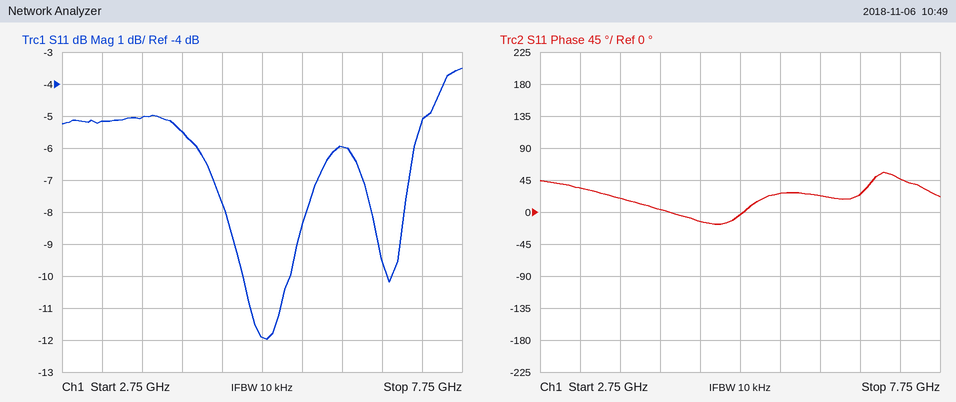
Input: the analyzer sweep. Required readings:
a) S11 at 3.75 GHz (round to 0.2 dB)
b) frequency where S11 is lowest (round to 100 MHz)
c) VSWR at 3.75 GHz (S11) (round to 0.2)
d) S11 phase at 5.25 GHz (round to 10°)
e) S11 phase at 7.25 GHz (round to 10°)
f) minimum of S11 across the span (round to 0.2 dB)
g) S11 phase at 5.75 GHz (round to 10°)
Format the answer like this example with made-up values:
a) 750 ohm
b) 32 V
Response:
a) -5.0 dB
b) 5.3 GHz
c) 3.6
d) 0°
e) 50°
f) -12.0 dB
g) 30°
